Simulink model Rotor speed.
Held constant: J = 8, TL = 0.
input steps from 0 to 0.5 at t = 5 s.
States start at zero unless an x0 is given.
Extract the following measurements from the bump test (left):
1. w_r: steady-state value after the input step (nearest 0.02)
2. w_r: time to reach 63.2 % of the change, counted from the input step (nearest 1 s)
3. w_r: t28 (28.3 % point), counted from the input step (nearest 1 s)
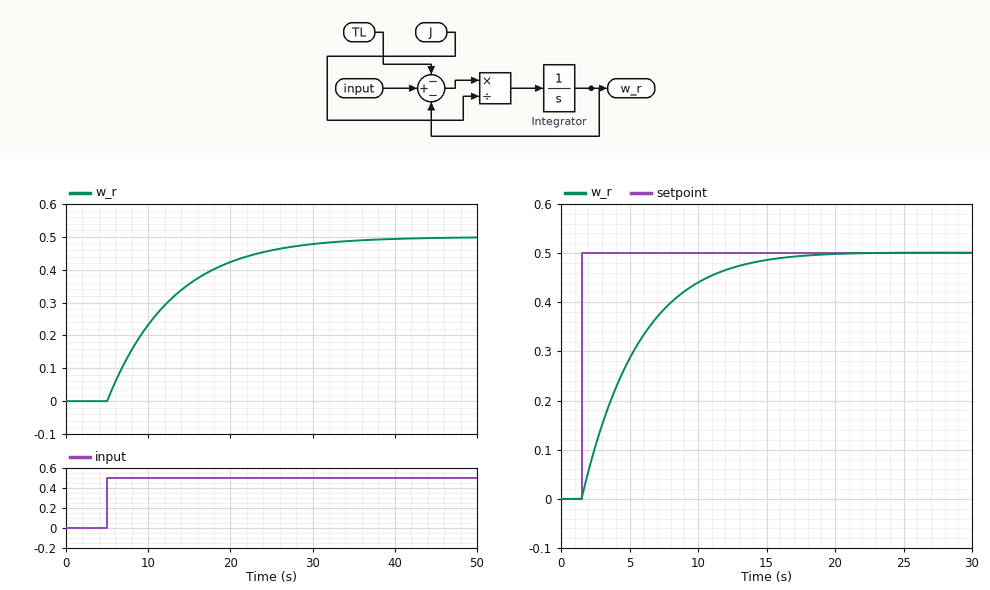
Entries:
0.50
8 s
3 s
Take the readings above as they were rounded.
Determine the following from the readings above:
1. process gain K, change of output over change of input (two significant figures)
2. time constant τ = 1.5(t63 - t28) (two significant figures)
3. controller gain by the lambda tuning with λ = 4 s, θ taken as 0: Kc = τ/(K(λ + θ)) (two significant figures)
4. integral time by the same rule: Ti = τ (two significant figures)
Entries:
1.0
7.5 s
1.9
7.5 s
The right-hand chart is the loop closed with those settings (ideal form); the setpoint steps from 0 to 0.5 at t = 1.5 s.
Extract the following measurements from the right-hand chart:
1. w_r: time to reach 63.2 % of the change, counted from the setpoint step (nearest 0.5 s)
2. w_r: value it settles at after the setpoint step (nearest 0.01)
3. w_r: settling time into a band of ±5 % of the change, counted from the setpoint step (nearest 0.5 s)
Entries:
4.0 s
0.50
11.5 s
